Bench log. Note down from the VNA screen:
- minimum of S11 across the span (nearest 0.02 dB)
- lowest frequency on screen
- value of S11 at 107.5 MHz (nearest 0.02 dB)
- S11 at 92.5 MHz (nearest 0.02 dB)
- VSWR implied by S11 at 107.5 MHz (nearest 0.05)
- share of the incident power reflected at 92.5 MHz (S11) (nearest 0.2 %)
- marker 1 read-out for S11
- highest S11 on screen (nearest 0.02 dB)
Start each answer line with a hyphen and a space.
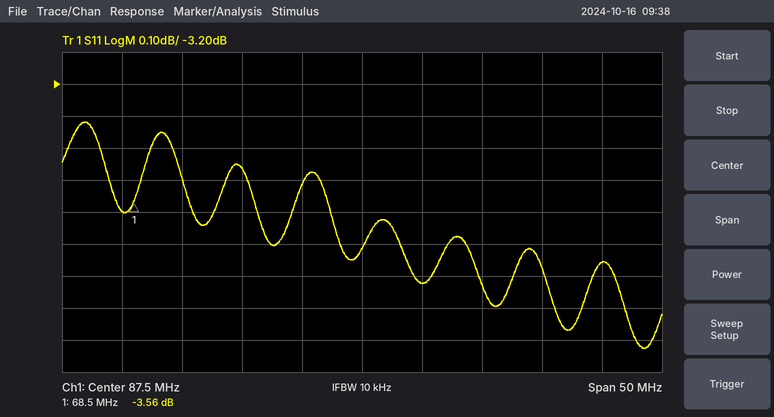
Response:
- -4.02 dB
- 62.5 MHz
- -3.76 dB
- -3.82 dB
- 4.70
- 41.4 %
- -3.56 dB
- -3.32 dB
